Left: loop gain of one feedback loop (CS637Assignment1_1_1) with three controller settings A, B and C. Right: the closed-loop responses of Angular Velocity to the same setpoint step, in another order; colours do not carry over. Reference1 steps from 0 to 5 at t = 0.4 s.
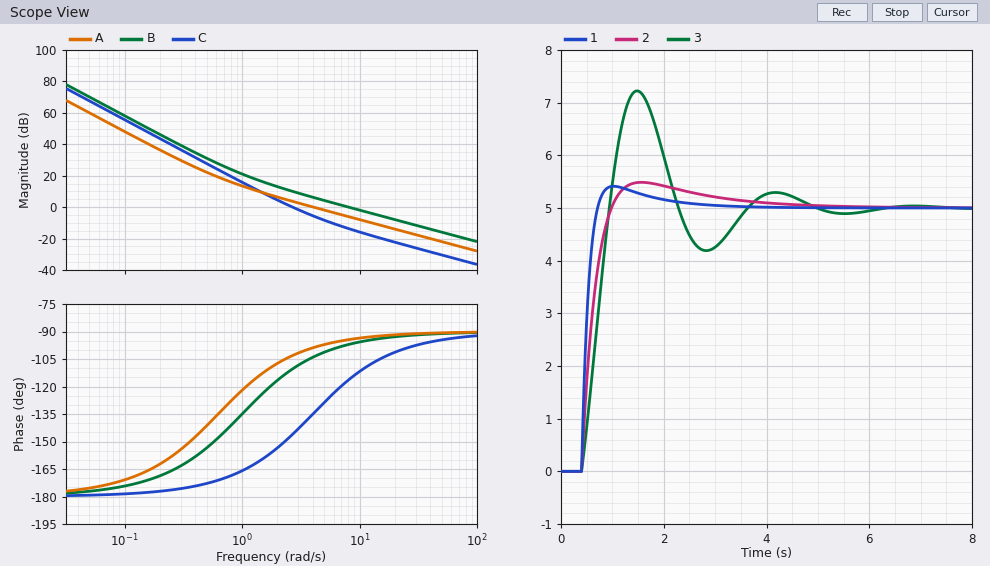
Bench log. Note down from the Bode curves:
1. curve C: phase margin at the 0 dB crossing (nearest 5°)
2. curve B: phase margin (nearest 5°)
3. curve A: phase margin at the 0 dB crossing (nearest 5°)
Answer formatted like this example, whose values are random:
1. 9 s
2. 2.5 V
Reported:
1. 35°
2. 85°
3. 80°
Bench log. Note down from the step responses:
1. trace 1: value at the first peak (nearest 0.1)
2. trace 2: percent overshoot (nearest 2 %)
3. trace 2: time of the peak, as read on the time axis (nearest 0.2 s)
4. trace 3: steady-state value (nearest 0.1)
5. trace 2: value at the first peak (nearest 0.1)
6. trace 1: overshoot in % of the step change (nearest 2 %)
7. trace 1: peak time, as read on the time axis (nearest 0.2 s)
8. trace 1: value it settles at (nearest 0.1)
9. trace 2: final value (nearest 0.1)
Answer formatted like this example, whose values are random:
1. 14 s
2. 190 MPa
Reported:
1. 5.4
2. 10 %
3. 1.6 s
4. 5.0
5. 5.5
6. 8 %
7. 1.0 s
8. 5.0
9. 5.0
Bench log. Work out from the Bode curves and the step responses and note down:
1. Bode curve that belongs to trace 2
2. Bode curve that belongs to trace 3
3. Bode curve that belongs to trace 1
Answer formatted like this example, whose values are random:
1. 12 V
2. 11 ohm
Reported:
1. A
2. C
3. B
